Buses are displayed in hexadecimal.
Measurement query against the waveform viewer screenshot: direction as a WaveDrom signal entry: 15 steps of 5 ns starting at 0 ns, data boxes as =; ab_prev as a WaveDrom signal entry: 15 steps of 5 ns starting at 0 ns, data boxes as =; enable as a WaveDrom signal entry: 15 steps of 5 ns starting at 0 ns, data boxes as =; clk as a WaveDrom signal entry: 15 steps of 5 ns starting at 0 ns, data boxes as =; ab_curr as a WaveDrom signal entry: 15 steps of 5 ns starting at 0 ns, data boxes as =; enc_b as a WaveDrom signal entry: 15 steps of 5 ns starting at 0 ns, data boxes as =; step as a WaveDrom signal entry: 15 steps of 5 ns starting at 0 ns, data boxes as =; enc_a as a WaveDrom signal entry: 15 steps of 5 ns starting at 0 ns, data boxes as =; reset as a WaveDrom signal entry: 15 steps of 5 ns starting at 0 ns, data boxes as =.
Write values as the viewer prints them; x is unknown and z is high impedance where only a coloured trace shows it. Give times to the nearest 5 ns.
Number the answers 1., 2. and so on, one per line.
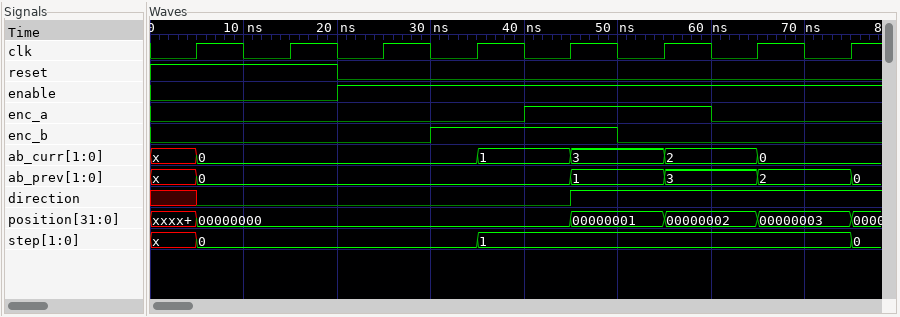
1. {name: 'direction', wave: 'x0.......1.....'}
2. {name: 'ab_prev', wave: 'x=.......=.=.=.', data: '0 1 3 2'}
3. {name: 'enable', wave: '0...1..........'}
4. {name: 'clk', wave: '010101010101010'}
5. {name: 'ab_curr', wave: 'x=.....=.=.=.=.', data: '0 1 3 2 0'}
6. {name: 'enc_b', wave: '0.....1...0....'}
7. {name: 'step', wave: 'x=.....=.......', data: '0 1'}
8. {name: 'enc_a', wave: '0.......1...0..'}
9. {name: 'reset', wave: '1...0..........'}
